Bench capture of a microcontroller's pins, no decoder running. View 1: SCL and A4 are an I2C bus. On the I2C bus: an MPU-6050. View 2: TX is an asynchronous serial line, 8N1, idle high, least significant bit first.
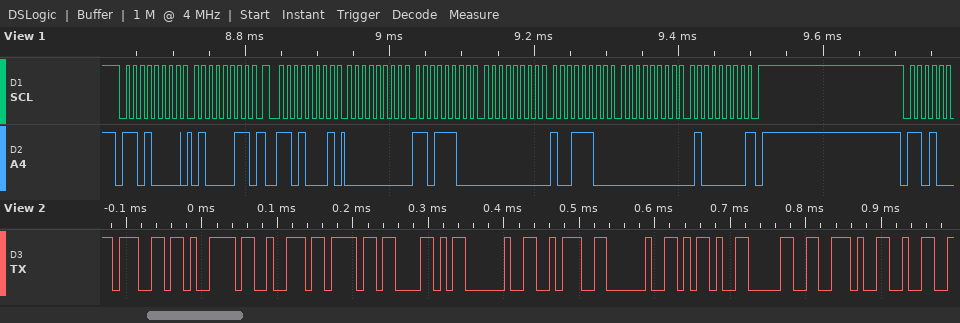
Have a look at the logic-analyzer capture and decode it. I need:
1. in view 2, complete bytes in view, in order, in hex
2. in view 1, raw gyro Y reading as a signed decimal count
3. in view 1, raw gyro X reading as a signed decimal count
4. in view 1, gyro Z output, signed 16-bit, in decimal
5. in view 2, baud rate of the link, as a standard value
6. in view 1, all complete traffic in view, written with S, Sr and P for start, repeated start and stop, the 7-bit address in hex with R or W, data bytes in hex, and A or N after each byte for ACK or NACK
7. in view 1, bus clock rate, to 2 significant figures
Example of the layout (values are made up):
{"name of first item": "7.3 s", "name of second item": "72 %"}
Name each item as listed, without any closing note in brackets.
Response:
{"in view 2, complete bytes in view, in order, in hex": "0x67 0x79 0x72 0x6F 0x58 0x20 0x3A 0x20 0x2D 0x30 0x2E 0x32", "in view 1, raw gyro Y reading as a signed decimal count": "156", "in view 1, raw gyro X reading as a signed decimal count": "220", "in view 1, gyro Z output, signed 16-bit, in decimal": "64", "in view 2, baud rate of the link, as a standard value": "115200 baud", "in view 1, all complete traffic in view, written with S, Sr and P for start, repeated start and stop, the 7-bit address in hex with R or W, data bytes in hex, and A or N after each byte for ACK or NACK": "S 68W A 43 A Sr 68R A 00 A DC A 00 A 9C A 00 A 40 N P", "in view 1, bus clock rate, to 2 significant figures": "100 kHz"}
